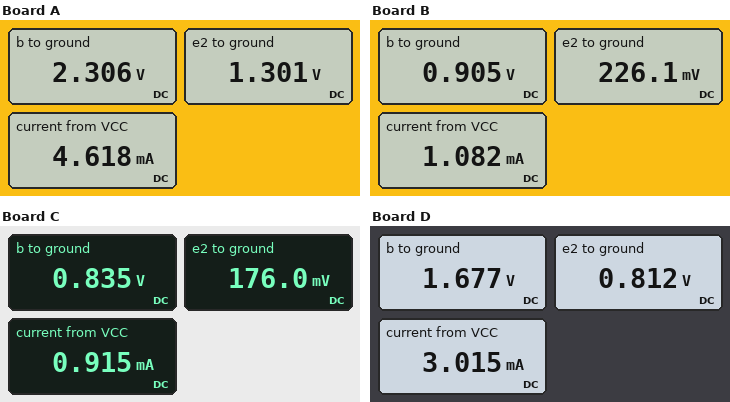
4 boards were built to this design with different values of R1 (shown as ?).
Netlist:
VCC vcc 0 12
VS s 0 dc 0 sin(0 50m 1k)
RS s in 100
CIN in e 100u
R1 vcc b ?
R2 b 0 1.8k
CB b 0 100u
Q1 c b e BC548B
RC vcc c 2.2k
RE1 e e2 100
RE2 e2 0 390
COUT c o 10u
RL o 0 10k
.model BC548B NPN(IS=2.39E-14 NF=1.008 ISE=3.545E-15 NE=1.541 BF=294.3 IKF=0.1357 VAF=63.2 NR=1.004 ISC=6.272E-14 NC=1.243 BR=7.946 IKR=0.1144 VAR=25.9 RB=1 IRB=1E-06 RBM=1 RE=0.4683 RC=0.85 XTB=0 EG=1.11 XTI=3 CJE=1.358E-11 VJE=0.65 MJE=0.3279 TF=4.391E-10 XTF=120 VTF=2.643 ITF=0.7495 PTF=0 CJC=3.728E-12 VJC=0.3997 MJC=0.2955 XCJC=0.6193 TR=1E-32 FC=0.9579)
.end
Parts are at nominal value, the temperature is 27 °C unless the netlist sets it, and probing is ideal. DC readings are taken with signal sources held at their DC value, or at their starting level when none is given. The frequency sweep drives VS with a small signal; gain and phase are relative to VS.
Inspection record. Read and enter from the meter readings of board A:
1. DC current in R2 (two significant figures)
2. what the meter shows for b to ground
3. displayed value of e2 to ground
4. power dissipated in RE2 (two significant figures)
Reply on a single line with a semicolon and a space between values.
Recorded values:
1.3 mA; 2.306 V; 1.301 V; 4.3 mW
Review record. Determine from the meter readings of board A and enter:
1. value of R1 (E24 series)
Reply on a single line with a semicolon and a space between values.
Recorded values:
7.5 kΩ
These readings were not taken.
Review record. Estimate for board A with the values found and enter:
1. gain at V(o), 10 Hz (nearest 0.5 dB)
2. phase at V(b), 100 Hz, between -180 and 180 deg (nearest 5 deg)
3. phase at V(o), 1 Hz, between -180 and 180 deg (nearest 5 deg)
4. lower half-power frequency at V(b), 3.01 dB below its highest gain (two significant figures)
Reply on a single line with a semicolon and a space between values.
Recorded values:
19.0 dB; -80 deg; 140 deg; 950 mHz
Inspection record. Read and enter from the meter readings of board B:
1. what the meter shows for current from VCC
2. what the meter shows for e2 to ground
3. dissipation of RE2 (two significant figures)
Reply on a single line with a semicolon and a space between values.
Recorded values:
1.082 mA; 226.1 mV; 130 µW
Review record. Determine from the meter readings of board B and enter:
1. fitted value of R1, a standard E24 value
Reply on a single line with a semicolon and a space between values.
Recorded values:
22 kΩ
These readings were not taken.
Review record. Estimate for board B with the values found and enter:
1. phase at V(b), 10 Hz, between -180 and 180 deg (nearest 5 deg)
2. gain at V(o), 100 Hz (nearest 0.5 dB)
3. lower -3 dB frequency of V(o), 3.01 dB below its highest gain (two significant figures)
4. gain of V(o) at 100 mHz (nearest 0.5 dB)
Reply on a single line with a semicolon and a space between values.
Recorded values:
-35 deg; 21.0 dB; 11 Hz; -42.0 dB
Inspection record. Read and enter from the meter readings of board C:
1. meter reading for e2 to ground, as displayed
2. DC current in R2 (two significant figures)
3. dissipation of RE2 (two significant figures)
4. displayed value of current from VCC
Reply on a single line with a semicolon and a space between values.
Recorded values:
176.0 mV; 460 µA; 79 µW; 0.915 mA
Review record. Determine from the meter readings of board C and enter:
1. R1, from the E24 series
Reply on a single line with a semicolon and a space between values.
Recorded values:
24 kΩ
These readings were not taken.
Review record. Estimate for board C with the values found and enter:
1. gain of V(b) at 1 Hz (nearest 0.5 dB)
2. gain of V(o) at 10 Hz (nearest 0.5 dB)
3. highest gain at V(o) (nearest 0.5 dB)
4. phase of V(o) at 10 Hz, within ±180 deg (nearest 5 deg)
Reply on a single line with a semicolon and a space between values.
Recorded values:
-54.0 dB; 17.0 dB; 20.5 dB; 55 deg
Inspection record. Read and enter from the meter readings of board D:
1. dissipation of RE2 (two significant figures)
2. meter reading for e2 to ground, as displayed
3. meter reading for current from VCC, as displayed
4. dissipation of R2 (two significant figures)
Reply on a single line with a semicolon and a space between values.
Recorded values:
1.7 mW; 0.812 V; 3.015 mA; 1.6 mW
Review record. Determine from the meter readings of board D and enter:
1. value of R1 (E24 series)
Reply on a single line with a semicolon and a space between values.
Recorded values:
11 kΩ
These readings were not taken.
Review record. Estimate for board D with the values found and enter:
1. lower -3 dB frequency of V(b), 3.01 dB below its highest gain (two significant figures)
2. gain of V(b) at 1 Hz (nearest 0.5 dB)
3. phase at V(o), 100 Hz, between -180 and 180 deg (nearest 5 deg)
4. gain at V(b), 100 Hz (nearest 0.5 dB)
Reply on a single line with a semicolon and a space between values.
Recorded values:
900 mHz; -52.5 dB; 10 deg; -66.5 dB
